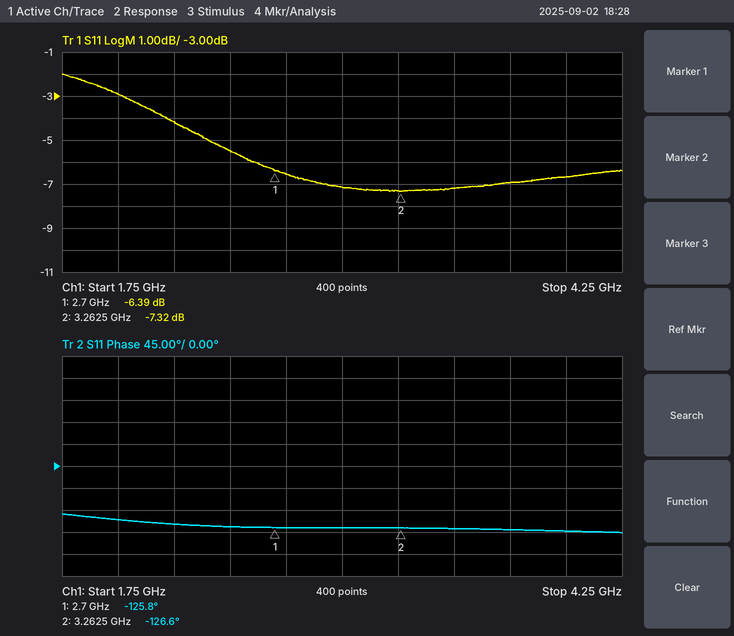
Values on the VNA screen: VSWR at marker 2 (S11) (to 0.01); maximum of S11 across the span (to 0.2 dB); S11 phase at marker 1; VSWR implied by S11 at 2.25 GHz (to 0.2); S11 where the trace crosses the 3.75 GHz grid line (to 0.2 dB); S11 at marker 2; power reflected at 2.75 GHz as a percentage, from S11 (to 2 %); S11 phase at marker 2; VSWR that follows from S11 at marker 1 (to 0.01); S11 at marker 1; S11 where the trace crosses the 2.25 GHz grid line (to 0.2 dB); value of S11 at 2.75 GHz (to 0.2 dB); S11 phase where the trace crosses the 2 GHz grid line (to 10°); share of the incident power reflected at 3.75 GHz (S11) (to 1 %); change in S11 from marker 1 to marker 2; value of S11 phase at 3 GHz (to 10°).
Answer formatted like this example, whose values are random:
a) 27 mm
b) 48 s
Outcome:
a) 2.51
b) -2.0 dB
c) -125.8°
d) 4.2
e) -7.0 dB
f) -7.32 dB
g) 22 %
h) -126.6°
i) 2.84
j) -6.39 dB
k) -4.2 dB
l) -6.6 dB
m) -110°
n) 20 %
o) -0.93 dB
p) -130°
